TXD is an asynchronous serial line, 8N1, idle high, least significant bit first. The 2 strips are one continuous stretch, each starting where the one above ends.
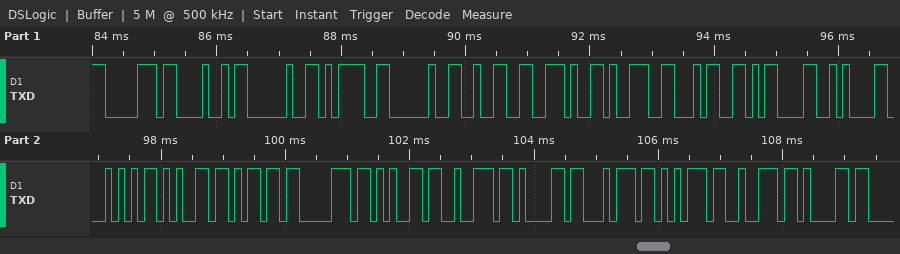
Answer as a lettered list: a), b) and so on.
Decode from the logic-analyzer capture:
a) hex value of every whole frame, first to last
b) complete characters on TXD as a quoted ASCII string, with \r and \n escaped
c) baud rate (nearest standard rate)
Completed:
a) 70 48 20 3D 20 32 2E 39 34 0D 0A 54 65 6D 70 65 72 61 74 75 72 61
b) "pH = 2.94\r\nTemperatura"
c) 9600 baud
